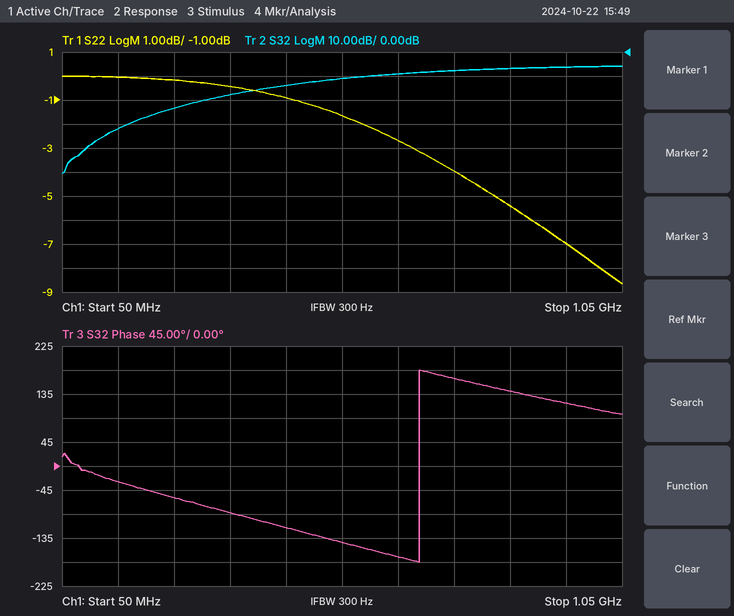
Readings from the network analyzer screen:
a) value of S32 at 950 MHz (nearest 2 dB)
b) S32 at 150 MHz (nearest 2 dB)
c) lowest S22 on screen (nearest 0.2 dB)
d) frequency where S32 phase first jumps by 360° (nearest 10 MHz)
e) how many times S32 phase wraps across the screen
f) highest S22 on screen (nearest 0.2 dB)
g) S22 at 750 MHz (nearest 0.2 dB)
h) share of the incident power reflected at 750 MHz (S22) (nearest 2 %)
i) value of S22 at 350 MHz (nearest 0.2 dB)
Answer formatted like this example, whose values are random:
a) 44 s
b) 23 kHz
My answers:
a) -6 dB
b) -32 dB
c) -8.6 dB
d) 690 MHz
e) 1
f) 0.0 dB
g) -4.0 dB
h) 40 %
i) -0.4 dB
